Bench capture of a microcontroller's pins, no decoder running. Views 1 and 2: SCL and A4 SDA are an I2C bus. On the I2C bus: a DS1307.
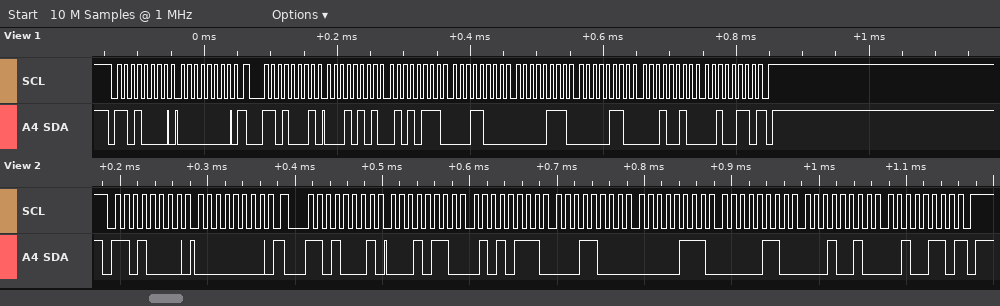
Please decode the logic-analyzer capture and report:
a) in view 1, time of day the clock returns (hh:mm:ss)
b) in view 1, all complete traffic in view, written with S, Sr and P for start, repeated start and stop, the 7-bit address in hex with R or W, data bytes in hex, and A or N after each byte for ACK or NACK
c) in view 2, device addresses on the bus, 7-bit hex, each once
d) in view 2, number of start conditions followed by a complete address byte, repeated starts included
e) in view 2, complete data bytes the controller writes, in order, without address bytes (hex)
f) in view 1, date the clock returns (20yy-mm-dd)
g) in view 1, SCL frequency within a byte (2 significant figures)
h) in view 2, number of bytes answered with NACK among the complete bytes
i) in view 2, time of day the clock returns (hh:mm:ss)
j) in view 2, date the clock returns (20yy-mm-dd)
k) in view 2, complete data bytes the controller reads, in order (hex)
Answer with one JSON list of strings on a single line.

["18:57:15", "S 68W A 00 A Sr 68R A 15 A 57 A 18 A 07 A 06 A 12 A 26 N P", "0x68", "2", "00", "2026-12-06", "100 kHz", "1", "18:57:16", "2026-12-06", "16 57 18 07 06 12 26"]
